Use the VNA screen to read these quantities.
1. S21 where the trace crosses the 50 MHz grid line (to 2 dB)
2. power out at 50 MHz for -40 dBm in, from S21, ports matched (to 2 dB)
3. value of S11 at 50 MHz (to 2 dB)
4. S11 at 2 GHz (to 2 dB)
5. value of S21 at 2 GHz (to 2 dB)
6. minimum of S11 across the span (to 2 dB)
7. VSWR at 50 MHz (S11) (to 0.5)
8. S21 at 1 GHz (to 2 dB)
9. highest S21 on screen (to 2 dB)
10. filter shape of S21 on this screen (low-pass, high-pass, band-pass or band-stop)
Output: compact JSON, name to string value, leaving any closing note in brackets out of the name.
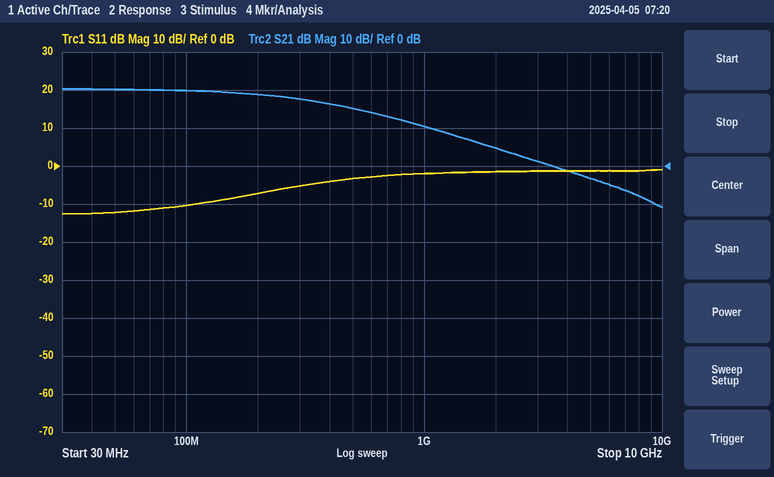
{"S21 where the trace crosses the 50 MHz grid line": "20 dB", "power out at 50 MHz for -40 dBm in, from S21, ports matched": "-20 dBm", "value of S11 at 50 MHz": "-12 dB", "S11 at 2 GHz": "-2 dB", "value of S21 at 2 GHz": "4 dB", "minimum of S11 across the span": "-12 dB", "VSWR at 50 MHz (S11)": "1.5", "S21 at 1 GHz": "10 dB", "highest S21 on screen": "20 dB", "filter shape of S21 on this screen": "low-pass"}
